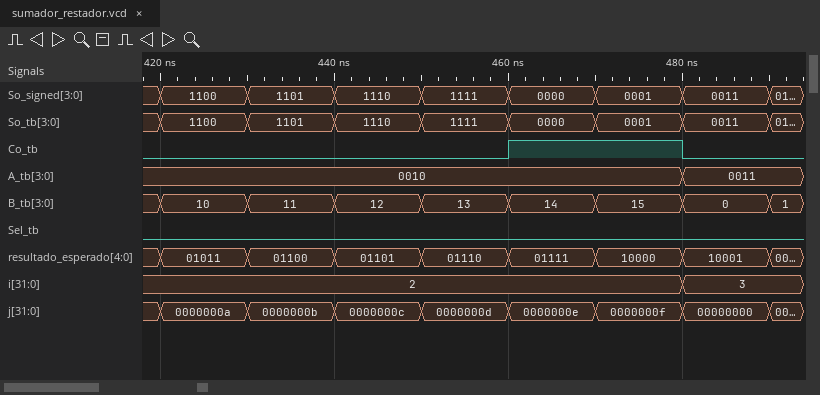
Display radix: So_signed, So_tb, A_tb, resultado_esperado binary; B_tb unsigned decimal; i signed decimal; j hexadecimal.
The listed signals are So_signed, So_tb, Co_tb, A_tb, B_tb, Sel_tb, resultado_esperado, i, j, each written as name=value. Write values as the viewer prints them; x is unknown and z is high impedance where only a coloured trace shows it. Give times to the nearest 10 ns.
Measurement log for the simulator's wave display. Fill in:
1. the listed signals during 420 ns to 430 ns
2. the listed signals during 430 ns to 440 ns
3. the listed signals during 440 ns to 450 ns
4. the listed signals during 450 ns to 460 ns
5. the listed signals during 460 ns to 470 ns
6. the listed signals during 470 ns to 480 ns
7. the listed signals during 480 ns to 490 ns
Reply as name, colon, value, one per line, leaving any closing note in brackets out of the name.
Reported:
the listed signals during 420 ns to 430 ns: So_signed=1100, So_tb=1100, Co_tb=0, A_tb=0010, B_tb=10, Sel_tb=0, resultado_esperado=01011, i=2, j=0000000a
the listed signals during 430 ns to 440 ns: So_signed=1101, So_tb=1101, Co_tb=0, A_tb=0010, B_tb=11, Sel_tb=0, resultado_esperado=01100, i=2, j=0000000b
the listed signals during 440 ns to 450 ns: So_signed=1110, So_tb=1110, Co_tb=0, A_tb=0010, B_tb=12, Sel_tb=0, resultado_esperado=01101, i=2, j=0000000c
the listed signals during 450 ns to 460 ns: So_signed=1111, So_tb=1111, Co_tb=0, A_tb=0010, B_tb=13, Sel_tb=0, resultado_esperado=01110, i=2, j=0000000d
the listed signals during 460 ns to 470 ns: So_signed=0000, So_tb=0000, Co_tb=1, A_tb=0010, B_tb=14, Sel_tb=0, resultado_esperado=01111, i=2, j=0000000e
the listed signals during 470 ns to 480 ns: So_signed=0001, So_tb=0001, Co_tb=1, A_tb=0010, B_tb=15, Sel_tb=0, resultado_esperado=10000, i=2, j=0000000f
the listed signals during 480 ns to 490 ns: So_signed=0011, So_tb=0011, Co_tb=0, A_tb=0011, B_tb=0, Sel_tb=0, resultado_esperado=10001, i=3, j=00000000
